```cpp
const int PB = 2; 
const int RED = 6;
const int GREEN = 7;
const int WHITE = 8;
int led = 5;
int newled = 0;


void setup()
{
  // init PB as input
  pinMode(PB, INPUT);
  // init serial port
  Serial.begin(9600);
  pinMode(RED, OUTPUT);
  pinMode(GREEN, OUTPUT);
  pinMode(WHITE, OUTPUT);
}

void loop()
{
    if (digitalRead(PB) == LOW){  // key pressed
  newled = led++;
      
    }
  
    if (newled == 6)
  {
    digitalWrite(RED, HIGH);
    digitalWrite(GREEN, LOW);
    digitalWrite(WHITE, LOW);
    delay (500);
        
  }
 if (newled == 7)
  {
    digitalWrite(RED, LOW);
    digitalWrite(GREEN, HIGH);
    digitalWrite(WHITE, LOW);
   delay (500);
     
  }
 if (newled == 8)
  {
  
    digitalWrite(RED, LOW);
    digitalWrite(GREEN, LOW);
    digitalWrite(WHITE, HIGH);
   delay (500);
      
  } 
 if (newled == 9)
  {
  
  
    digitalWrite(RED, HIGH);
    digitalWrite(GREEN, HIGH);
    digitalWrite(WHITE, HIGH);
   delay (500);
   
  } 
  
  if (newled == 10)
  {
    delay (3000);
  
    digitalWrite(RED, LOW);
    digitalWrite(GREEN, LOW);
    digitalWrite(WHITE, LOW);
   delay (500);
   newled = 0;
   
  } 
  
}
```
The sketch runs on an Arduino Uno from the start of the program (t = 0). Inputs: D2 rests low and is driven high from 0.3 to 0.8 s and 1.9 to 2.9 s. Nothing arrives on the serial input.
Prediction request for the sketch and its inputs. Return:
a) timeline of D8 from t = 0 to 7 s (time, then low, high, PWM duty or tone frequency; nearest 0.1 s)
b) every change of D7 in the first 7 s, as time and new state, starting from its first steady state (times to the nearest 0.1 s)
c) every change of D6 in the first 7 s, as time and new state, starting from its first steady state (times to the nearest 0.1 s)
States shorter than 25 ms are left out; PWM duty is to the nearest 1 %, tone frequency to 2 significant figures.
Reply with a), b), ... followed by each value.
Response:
a) 0 s low; 1.5 s high; 6.5 s low
b) 0 s low; 1 s high; 1.5 s low; 3 s high; 6.5 s low
c) 0 s high; 1 s low; 3 s high; 6.5 s low
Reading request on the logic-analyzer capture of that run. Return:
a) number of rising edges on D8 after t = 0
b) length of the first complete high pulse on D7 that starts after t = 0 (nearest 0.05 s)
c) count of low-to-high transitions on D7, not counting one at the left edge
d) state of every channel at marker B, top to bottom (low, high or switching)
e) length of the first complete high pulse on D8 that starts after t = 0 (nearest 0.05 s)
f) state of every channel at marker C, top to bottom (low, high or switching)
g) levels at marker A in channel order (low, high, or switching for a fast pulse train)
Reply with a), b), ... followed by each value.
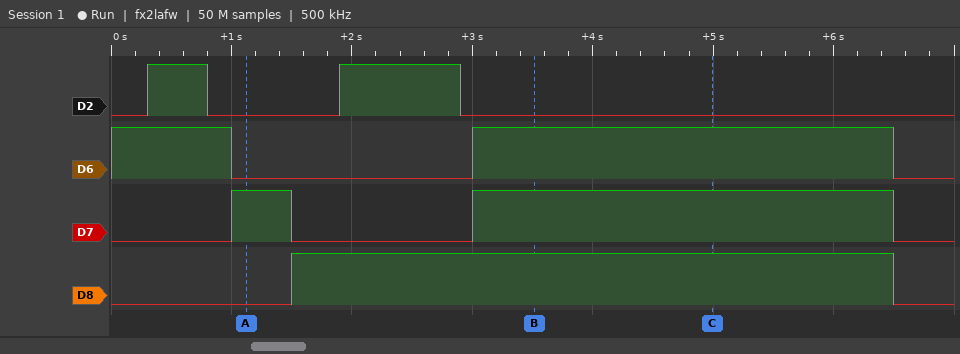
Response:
a) 1
b) 0.50 s
c) 2
d) D2 low, D6 high, D7 high, D8 high
e) 5.00 s
f) D2 low, D6 high, D7 high, D8 high
g) D2 low, D6 low, D7 high, D8 low
